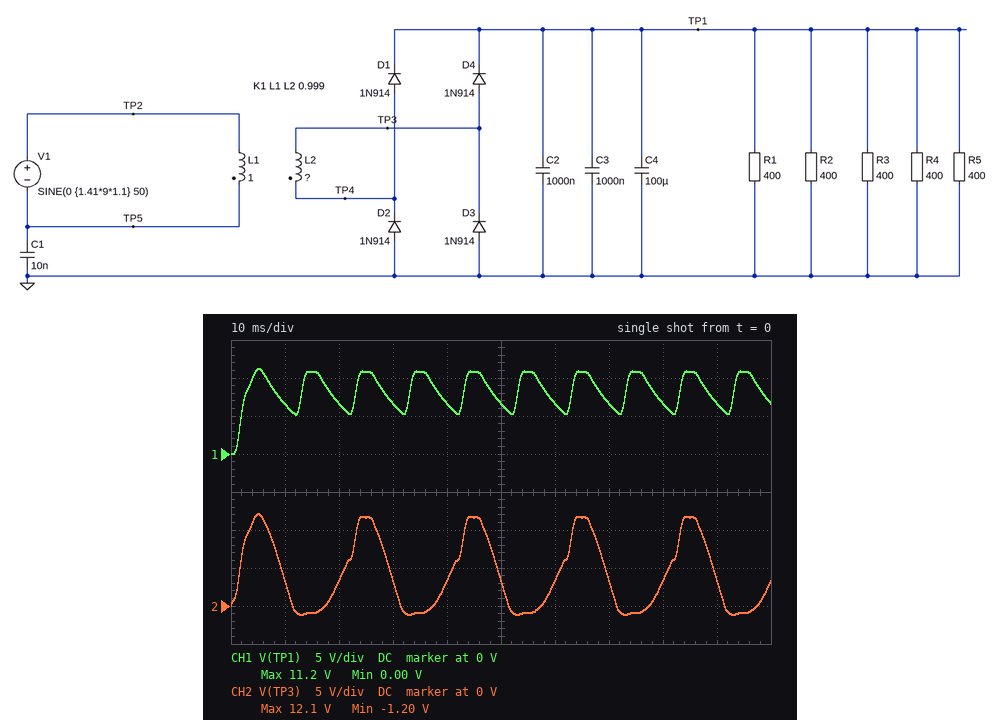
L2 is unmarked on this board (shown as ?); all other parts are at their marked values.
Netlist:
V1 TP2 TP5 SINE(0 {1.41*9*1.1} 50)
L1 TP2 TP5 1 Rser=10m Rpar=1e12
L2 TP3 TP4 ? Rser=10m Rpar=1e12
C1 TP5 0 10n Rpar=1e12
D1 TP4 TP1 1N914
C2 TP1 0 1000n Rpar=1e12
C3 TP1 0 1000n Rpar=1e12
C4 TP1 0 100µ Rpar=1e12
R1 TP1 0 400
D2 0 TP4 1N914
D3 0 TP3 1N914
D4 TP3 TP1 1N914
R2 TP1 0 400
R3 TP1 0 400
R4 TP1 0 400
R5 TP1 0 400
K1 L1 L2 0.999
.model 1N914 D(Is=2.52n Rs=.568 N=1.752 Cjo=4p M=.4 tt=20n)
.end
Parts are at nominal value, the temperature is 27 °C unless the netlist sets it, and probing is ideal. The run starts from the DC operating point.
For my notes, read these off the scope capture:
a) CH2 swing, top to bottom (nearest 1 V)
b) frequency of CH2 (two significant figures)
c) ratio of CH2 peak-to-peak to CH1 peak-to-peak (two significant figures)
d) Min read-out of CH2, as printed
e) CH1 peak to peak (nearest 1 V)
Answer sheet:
13 V
50 Hz
1.2
-1.20 V
11 V
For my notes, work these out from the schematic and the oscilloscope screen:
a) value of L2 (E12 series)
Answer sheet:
820 mH
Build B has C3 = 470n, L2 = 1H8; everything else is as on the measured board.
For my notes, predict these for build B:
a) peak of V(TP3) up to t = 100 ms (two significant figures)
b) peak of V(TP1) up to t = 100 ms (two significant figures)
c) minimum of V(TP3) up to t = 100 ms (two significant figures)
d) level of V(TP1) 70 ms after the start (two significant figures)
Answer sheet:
20 V
19 V
-1.4 V
10 V
